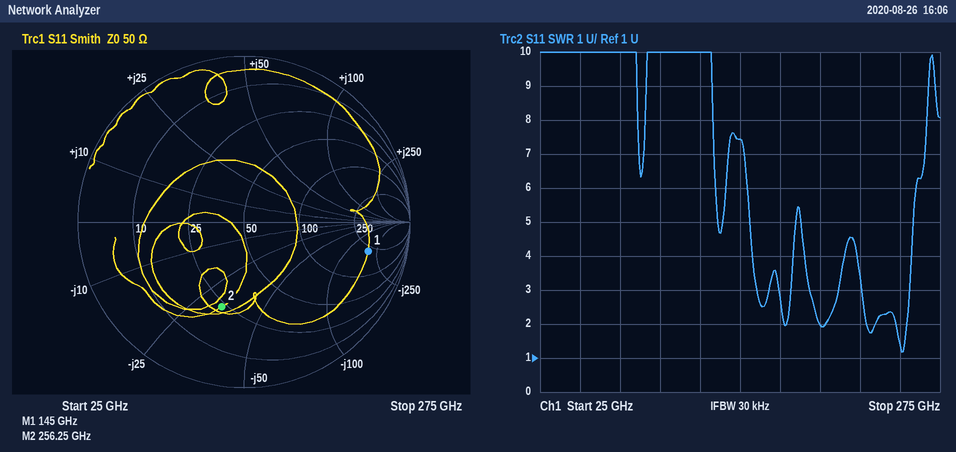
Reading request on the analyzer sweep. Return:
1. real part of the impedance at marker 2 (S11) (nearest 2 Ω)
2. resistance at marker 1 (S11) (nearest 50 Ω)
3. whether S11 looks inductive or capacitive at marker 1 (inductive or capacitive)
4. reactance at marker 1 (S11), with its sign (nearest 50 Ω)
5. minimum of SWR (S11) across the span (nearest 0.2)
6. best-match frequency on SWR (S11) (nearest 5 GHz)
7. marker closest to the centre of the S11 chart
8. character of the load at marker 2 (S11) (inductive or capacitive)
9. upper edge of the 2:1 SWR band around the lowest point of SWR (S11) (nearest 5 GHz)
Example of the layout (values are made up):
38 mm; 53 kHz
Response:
24 Ω; 200 Ω; capacitive; -200 Ω; 1.2; 250 GHz; marker 2; capacitive; 255 GHz
